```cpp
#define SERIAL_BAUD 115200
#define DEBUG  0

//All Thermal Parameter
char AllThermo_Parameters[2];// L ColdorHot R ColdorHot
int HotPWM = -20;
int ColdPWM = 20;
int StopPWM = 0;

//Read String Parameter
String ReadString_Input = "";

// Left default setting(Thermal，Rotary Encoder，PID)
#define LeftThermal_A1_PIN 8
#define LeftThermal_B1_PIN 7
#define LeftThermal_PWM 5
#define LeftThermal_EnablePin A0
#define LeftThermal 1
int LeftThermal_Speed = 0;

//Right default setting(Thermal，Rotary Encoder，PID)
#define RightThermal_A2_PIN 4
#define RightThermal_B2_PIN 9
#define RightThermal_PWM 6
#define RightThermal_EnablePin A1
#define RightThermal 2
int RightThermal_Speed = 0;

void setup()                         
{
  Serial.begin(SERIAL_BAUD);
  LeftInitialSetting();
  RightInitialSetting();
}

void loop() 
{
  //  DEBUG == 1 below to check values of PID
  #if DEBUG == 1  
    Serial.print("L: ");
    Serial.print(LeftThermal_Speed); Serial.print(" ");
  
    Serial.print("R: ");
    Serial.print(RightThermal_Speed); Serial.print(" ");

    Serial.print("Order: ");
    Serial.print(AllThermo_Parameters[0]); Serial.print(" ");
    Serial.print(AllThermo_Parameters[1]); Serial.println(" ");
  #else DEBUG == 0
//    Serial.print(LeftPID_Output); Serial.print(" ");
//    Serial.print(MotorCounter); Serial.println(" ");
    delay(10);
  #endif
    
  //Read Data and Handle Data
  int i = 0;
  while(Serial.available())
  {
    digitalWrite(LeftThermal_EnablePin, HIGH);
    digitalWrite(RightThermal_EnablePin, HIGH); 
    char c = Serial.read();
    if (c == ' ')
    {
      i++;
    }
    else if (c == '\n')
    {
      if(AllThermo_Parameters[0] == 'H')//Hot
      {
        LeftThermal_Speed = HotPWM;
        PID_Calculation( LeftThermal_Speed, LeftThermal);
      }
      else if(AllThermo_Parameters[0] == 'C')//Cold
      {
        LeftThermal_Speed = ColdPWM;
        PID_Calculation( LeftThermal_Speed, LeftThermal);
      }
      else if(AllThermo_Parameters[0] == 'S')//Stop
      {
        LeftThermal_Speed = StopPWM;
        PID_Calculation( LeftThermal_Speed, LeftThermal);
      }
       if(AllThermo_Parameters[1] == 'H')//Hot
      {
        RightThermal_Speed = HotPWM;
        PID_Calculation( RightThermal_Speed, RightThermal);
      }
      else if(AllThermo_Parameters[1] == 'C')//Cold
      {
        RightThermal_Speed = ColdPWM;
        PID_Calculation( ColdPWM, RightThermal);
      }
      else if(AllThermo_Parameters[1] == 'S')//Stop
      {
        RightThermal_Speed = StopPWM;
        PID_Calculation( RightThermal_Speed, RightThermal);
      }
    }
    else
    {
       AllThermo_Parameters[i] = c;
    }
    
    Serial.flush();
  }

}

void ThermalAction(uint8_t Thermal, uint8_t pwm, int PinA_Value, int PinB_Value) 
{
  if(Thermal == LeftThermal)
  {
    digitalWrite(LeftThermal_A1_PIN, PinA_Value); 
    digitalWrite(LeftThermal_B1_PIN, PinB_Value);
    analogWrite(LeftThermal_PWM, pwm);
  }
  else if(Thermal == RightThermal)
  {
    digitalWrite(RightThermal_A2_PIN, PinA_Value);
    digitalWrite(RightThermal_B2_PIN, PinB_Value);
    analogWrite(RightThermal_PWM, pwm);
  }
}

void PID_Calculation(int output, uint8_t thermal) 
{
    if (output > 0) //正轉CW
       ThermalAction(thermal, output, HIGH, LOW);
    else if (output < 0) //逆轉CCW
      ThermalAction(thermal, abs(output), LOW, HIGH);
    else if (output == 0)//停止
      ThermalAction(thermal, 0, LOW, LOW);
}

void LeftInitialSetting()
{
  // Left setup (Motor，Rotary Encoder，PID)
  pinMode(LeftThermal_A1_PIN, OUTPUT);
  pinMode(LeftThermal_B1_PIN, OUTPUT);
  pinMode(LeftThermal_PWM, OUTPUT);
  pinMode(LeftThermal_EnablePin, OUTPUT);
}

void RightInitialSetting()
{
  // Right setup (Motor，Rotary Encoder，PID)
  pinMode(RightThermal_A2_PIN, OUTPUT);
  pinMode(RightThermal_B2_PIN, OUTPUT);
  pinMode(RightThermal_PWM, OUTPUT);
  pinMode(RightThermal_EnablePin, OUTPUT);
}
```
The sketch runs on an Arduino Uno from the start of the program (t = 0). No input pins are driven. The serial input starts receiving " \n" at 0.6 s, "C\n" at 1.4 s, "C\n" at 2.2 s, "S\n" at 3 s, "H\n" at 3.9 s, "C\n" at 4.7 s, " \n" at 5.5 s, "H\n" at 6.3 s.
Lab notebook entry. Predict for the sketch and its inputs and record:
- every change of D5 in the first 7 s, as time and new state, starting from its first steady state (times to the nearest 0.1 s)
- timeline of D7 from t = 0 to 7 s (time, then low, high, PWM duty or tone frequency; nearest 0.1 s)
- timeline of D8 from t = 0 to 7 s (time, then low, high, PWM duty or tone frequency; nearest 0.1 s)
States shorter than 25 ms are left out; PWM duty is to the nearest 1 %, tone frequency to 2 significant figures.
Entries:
0 s low; 1.4 s PWM 8 %; 3 s low; 3.9 s PWM 8 %
0 s low; 3.9 s high; 4.7 s low; 6.3 s high
0 s low; 1.4 s high; 3 s low; 4.7 s high; 6.3 s low
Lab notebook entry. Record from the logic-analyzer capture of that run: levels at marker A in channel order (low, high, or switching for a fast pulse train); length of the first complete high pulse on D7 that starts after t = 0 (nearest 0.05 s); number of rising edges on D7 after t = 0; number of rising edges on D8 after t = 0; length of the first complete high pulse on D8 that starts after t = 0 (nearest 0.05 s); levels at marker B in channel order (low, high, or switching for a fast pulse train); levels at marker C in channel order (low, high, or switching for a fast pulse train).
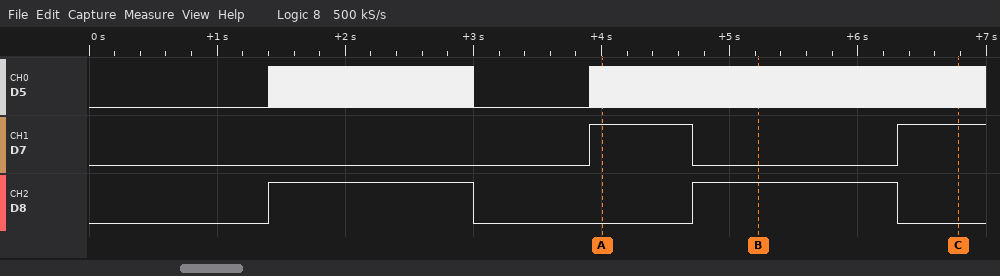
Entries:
D5 switching, D7 high, D8 low
0.80 s
2
2
1.60 s
D5 switching, D7 low, D8 high
D5 switching, D7 high, D8 low
